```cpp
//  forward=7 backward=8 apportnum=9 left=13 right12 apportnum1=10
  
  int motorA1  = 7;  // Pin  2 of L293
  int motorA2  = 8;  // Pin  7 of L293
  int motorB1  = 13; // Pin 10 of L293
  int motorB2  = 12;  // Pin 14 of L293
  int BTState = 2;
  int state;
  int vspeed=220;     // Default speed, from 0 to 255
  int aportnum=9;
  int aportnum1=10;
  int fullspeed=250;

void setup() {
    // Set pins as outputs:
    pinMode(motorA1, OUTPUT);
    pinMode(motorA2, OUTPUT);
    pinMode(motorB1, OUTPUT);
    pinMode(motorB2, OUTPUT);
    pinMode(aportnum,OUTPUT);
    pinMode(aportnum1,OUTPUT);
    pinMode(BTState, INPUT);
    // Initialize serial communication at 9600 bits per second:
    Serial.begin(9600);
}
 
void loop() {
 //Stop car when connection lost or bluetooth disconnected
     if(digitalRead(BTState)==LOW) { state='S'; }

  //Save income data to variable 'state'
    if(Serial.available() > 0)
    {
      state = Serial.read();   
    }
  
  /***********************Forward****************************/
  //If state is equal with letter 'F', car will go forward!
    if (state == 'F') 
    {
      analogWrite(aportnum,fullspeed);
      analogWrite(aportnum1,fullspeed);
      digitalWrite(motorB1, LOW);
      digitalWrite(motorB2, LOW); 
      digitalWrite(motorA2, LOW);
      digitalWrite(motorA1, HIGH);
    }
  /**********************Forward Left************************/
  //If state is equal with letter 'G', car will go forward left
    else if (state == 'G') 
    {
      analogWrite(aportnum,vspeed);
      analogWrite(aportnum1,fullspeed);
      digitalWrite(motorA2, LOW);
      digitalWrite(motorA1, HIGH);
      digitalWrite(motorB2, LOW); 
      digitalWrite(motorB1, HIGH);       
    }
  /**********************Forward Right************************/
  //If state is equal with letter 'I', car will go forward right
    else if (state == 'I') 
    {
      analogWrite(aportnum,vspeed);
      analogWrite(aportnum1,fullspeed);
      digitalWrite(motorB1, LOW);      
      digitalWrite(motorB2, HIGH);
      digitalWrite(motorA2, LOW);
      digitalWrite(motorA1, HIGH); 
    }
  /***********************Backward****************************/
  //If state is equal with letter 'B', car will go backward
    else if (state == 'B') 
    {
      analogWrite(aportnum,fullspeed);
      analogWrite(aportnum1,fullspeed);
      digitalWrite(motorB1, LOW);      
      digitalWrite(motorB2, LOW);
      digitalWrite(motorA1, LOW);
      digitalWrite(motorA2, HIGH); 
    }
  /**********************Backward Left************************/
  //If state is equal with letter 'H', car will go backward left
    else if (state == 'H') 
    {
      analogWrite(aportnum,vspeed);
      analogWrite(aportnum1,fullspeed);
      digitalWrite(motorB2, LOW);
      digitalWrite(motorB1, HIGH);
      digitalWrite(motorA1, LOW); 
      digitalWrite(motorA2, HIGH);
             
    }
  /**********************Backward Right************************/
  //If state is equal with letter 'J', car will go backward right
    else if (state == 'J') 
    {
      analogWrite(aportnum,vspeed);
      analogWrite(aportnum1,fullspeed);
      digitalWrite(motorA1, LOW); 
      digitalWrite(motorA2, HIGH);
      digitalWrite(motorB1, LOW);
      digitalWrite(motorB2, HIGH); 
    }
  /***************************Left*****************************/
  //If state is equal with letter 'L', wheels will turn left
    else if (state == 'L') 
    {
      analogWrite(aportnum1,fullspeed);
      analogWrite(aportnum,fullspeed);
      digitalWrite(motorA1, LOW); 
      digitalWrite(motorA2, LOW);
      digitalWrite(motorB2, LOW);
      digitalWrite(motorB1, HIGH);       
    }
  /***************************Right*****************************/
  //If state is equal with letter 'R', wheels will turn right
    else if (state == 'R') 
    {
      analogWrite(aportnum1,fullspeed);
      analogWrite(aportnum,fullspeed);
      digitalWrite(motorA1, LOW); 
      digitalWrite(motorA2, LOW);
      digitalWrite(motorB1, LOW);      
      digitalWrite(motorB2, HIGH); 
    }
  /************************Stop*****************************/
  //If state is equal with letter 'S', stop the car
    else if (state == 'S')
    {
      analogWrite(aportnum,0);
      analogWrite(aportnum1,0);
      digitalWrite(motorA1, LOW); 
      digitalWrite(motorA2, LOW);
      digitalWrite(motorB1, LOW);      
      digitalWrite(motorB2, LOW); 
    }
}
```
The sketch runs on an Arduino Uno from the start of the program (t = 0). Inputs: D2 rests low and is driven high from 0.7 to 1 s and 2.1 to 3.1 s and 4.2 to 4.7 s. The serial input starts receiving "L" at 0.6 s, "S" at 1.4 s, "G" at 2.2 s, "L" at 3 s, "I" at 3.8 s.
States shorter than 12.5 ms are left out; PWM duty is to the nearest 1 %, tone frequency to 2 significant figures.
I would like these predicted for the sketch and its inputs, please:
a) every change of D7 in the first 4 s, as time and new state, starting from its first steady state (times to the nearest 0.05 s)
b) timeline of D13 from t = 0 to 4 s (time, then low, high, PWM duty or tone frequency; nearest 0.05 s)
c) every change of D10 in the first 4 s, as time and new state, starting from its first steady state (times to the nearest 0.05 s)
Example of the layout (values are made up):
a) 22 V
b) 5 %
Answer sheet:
a) 0 s low; 2.2 s high; 3 s low
b) 0 s low; 2.2 s high; 3.1 s low
c) 0 s low; 2.2 s PWM 98 %; 3.1 s low
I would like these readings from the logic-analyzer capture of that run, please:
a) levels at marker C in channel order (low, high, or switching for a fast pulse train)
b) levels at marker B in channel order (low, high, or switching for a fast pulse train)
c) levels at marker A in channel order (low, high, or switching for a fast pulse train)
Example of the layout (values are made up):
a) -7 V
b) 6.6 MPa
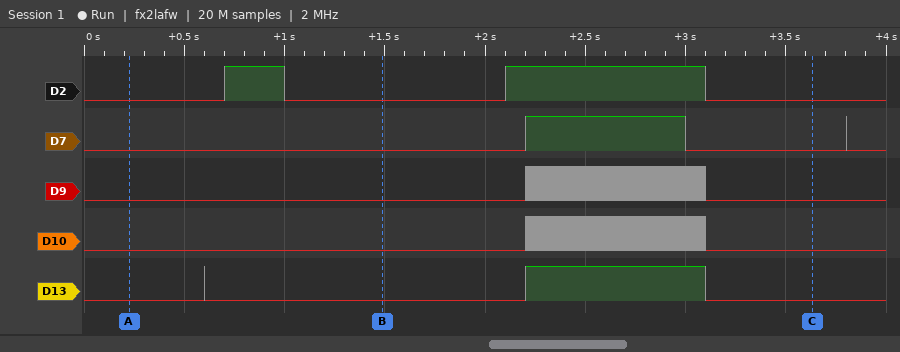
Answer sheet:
a) D2 low, D7 low, D9 low, D10 low, D13 low
b) D2 low, D7 low, D9 low, D10 low, D13 low
c) D2 low, D7 low, D9 low, D10 low, D13 low
